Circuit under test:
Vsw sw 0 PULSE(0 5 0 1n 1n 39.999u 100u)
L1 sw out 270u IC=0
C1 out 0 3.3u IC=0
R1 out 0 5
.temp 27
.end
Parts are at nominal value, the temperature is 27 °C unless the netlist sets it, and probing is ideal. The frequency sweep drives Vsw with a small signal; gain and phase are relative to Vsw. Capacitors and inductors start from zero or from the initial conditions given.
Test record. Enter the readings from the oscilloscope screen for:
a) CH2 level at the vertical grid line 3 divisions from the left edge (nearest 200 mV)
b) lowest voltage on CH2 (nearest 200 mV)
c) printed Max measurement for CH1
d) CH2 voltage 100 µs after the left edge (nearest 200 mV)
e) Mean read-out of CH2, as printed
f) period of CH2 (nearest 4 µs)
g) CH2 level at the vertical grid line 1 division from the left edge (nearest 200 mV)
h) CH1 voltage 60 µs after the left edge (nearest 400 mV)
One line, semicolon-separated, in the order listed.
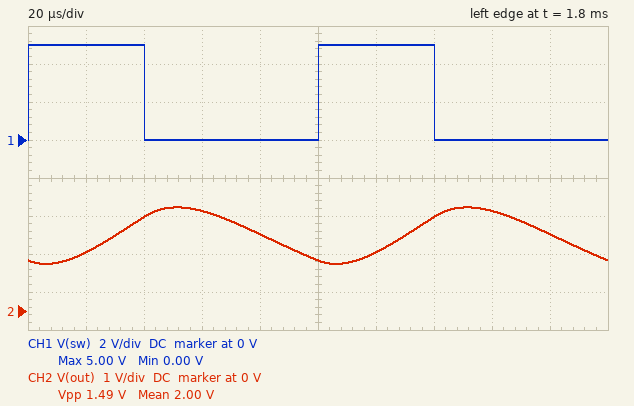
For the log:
2.6 V; 1.2 V; 5.00 V; 1.4 V; 2.00 V; 100 µs; 1.6 V; 0 V
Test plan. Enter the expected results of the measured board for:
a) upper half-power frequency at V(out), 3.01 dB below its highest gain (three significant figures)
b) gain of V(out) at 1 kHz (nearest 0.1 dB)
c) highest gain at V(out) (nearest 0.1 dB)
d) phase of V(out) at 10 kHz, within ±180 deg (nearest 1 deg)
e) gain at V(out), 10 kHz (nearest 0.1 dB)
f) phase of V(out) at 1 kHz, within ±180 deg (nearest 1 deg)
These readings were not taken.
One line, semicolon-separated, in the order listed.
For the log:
3.95 kHz; -0.2 dB; 0 dB; -127 deg; -12.5 dB; -19 deg
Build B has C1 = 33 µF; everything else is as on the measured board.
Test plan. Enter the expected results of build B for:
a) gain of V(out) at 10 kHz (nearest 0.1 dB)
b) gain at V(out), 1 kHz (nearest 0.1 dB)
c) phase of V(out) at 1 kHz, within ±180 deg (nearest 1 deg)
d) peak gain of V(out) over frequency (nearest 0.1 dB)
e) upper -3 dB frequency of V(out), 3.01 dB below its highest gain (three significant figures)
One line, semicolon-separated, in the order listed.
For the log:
-30.7 dB; 2.7 dB; -28 deg; 5.2 dB; 1.98 kHz
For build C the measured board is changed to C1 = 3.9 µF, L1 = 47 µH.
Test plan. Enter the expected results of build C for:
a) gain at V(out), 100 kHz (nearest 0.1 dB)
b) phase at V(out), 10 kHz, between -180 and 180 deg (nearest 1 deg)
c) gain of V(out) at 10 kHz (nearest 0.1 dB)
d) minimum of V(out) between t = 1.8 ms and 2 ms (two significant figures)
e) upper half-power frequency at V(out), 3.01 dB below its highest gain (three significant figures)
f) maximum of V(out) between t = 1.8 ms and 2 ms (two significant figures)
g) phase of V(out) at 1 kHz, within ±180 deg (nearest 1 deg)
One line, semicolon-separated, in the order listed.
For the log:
-37.1 dB; -65 deg; 3.7 dB; -2.2 V; 14.0 kHz; 7.0 V; -3 deg
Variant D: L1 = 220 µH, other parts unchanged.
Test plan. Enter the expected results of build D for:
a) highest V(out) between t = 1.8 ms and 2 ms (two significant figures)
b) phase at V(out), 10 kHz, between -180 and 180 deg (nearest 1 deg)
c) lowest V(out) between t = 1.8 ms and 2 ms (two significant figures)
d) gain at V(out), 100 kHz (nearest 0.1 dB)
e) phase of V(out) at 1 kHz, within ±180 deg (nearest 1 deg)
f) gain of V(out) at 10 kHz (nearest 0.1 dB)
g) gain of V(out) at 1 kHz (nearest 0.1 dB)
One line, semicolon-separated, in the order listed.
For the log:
2.9 V; -124 deg; 1.0 V; -49.2 dB; -16 deg; -10.5 dB; -0.1 dB
